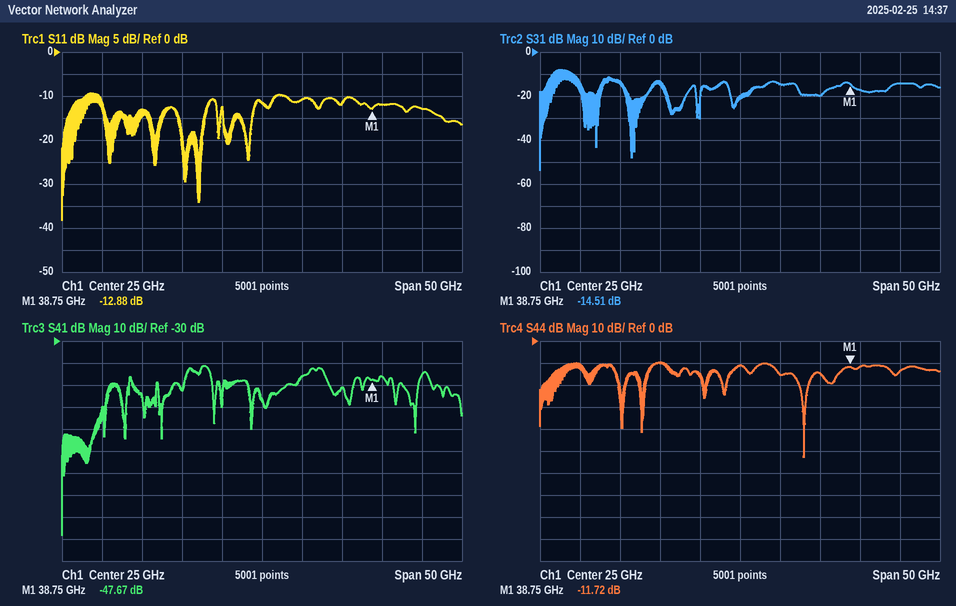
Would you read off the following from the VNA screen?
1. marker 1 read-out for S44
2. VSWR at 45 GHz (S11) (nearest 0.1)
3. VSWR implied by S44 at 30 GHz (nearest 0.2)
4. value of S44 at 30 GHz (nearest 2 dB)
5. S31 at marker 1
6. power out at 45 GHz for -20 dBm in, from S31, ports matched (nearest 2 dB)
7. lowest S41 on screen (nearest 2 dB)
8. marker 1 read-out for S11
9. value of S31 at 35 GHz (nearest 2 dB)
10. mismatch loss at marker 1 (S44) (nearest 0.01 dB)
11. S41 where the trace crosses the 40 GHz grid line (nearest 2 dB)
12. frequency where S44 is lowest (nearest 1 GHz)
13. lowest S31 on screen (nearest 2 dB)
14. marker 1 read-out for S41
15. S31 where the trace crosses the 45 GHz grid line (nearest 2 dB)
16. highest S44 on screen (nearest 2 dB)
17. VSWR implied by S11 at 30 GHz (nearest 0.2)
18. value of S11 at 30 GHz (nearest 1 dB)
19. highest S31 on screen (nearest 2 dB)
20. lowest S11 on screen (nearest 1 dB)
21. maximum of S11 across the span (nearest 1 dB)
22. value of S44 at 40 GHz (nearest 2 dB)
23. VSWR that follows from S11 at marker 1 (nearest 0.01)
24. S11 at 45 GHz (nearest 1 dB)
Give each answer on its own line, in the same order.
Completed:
-11.72 dB
1.6
1.4
-16 dB
-14.51 dB
-34 dBm
-118 dB
-12.88 dB
-20 dB
0.30 dB
-46 dB
33 GHz
-54 dB
-47.67 dB
-14 dB
-10 dB
1.8
-11 dB
-8 dB
-38 dB
-9 dB
-12 dB
1.59
-13 dB
